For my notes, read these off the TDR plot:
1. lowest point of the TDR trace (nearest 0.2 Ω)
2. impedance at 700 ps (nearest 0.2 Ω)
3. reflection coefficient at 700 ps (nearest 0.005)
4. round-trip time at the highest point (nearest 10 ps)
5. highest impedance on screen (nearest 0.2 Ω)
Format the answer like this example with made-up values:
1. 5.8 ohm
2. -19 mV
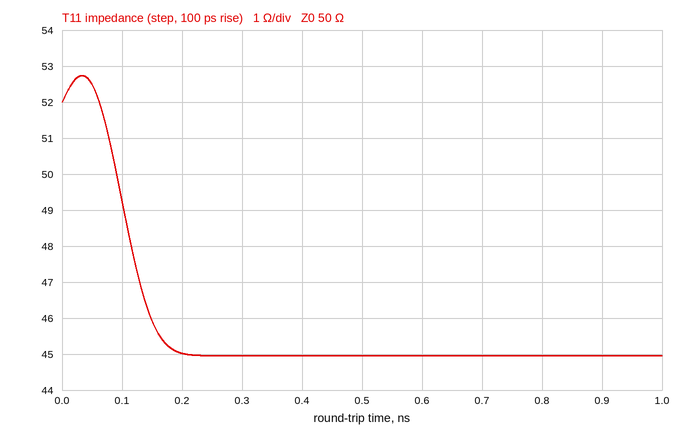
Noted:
1. 45.0 Ω
2. 45.0 Ω
3. -0.055
4. 30 ps
5. 52.8 Ω
